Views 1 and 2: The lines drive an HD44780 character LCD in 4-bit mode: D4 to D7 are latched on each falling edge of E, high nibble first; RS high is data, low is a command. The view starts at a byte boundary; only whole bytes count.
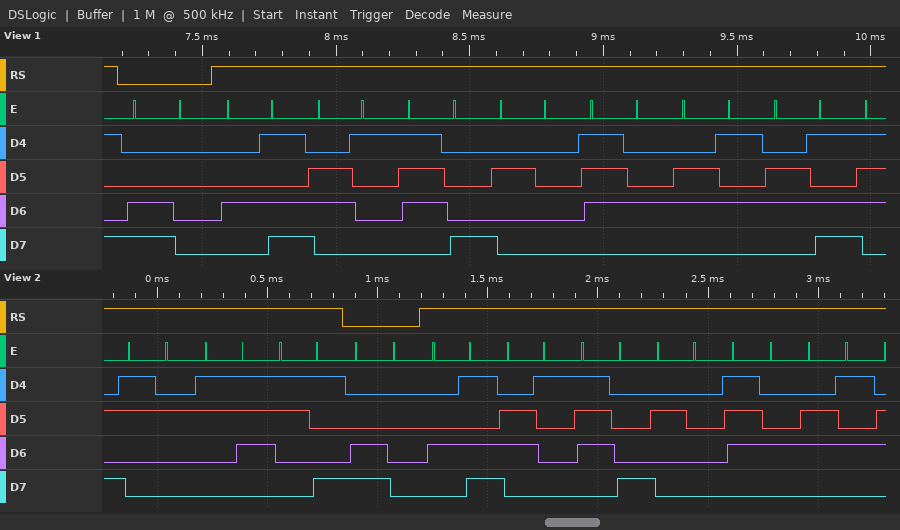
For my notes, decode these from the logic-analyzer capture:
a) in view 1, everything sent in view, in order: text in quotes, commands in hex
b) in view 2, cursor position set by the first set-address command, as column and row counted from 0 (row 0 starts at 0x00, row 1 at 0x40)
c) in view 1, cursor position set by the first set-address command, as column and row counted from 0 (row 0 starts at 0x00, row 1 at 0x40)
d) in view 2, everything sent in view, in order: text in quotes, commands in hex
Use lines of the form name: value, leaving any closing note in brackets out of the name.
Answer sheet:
in view 1, everything sent in view, in order: text in quotes, commands in hex: 0xC0 "Max tem"
in view 2, cursor position set by the first set-address command, as column and row counted from 0: column 0, row 1
in view 1, cursor position set by the first set-address command, as column and row counted from 0: column 0, row 1
in view 2, everything sent in view, in order: text in quotes, commands in hex: "279" 0xC0 "Max te"
